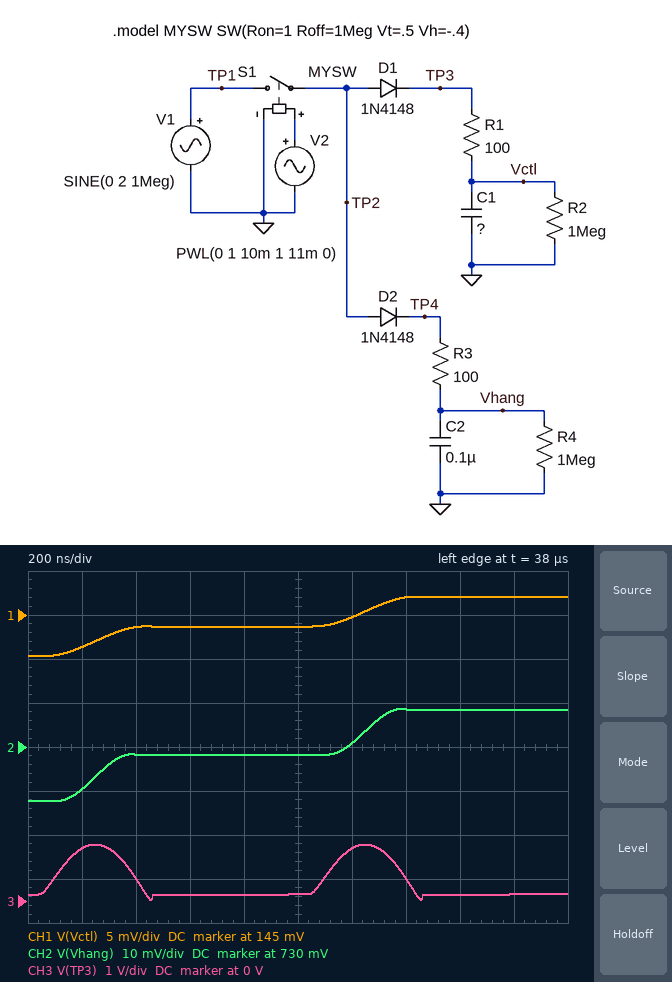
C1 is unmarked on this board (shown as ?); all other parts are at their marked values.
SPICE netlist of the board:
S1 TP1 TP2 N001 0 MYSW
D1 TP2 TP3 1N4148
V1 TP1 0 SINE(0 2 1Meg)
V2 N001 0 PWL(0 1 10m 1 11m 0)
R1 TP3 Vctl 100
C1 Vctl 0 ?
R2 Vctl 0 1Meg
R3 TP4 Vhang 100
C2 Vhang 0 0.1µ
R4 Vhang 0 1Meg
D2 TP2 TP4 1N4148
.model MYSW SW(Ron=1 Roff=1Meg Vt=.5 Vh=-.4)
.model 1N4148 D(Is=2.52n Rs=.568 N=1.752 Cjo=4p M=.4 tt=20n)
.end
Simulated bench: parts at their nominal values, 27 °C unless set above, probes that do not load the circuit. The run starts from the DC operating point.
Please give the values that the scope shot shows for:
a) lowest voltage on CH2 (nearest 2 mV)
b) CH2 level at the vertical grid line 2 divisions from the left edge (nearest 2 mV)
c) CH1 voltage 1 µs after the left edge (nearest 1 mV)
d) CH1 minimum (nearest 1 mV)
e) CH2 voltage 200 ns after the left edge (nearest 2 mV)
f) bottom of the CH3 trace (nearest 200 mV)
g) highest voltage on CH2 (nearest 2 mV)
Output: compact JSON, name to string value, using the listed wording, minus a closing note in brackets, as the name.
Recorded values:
{"lowest voltage on CH2": "718 mV", "CH2 level at the vertical grid line 2 divisions from the left edge": "728 mV", "CH1 voltage 1 µs after the left edge": "144 mV", "CH1 minimum": "140 mV", "CH2 voltage 200 ns after the left edge": "720 mV", "bottom of the CH3 trace": "0 V", "highest voltage on CH2": "738 mV"}
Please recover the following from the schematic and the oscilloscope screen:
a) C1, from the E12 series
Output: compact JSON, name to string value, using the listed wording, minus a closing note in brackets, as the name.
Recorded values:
{"C1, from the E12 series": "820 nF"}
